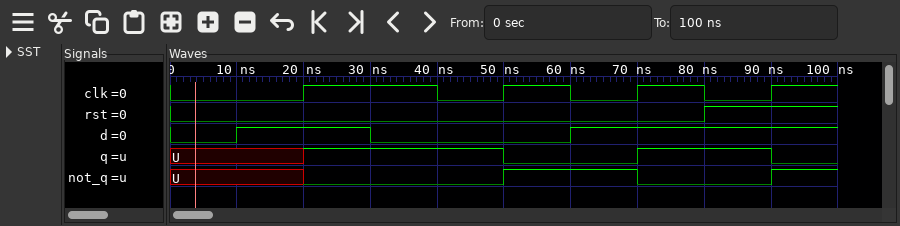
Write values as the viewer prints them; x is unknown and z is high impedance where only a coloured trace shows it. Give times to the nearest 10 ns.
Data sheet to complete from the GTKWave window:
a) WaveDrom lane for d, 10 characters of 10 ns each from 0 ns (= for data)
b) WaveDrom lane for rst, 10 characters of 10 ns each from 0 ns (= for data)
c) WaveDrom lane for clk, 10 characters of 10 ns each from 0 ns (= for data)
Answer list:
{name: 'd', wave: '01.0..1...'}
{name: 'rst', wave: '0.......1.'}
{name: 'clk', wave: '0.1.010101'}
